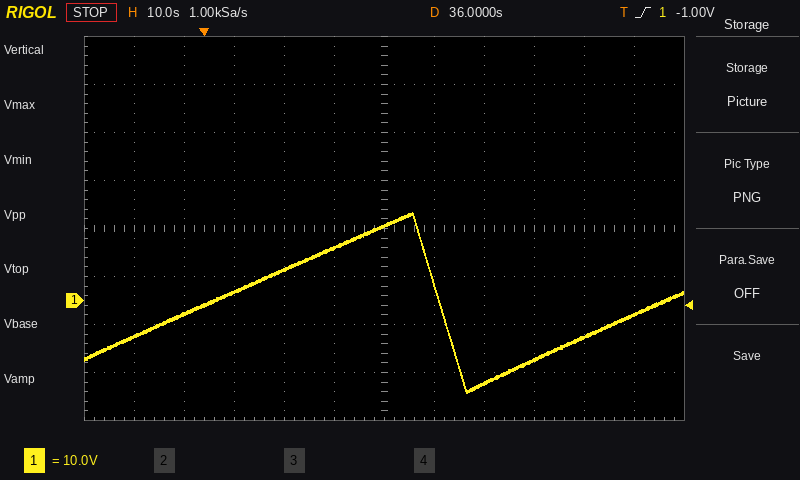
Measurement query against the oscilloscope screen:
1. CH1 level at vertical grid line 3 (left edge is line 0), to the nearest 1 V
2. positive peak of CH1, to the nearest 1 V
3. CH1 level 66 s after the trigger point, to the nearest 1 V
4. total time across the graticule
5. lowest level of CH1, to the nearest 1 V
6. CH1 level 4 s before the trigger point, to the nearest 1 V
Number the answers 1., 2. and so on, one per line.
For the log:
1. 2 V
2. 18 V
3. -12 V
4. 120 s
5. -19 V
6. -3 V
